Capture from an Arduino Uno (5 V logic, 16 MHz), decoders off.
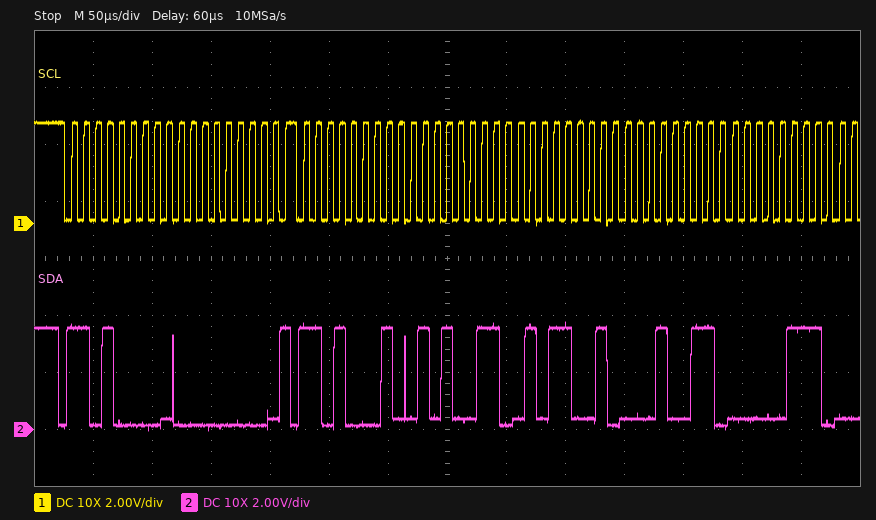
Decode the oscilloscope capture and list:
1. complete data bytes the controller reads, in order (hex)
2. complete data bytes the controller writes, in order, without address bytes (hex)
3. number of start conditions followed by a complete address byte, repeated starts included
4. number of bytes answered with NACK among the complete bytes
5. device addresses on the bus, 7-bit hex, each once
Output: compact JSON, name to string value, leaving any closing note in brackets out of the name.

{"complete data bytes the controller reads, in order": "53 59 13 07", "complete data bytes the controller writes, in order, without address bytes": "00", "number of start conditions followed by a complete address byte, repeated starts included": "2", "number of bytes answered with NACK among the complete bytes": "0", "device addresses on the bus, 7-bit hex, each once": "0x68"}
